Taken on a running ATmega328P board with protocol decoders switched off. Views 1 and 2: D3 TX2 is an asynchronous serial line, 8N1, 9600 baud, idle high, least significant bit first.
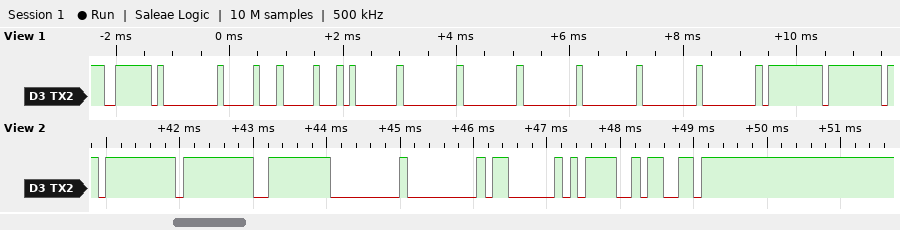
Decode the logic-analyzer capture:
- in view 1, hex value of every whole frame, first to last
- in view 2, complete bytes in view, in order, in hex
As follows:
7E 00 10 10 01 00 00 00 00 00 00 FF FF
0xFF 0xFF 0xFE 0x00 0x00 0x03 0x3D 0xB3
